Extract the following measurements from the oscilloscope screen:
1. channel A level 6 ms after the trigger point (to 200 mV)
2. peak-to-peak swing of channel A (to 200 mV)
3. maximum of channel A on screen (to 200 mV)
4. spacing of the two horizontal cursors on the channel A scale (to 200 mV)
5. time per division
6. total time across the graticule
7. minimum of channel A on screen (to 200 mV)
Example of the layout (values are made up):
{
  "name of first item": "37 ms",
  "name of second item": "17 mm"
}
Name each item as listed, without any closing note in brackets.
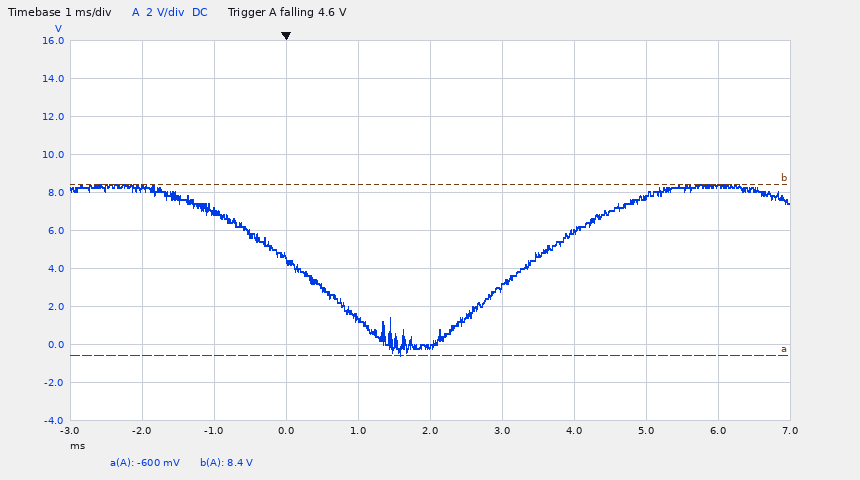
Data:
{
  "channel A level 6 ms after the trigger point": "8.4 V",
  "peak-to-peak swing of channel A": "9.0 V",
  "maximum of channel A on screen": "8.4 V",
  "spacing of the two horizontal cursors on the channel A scale": "9.0 V",
  "time per division": "1 ms",
  "total time across the graticule": "10 ms",
  "minimum of channel A on screen": "-600 mV"
}
